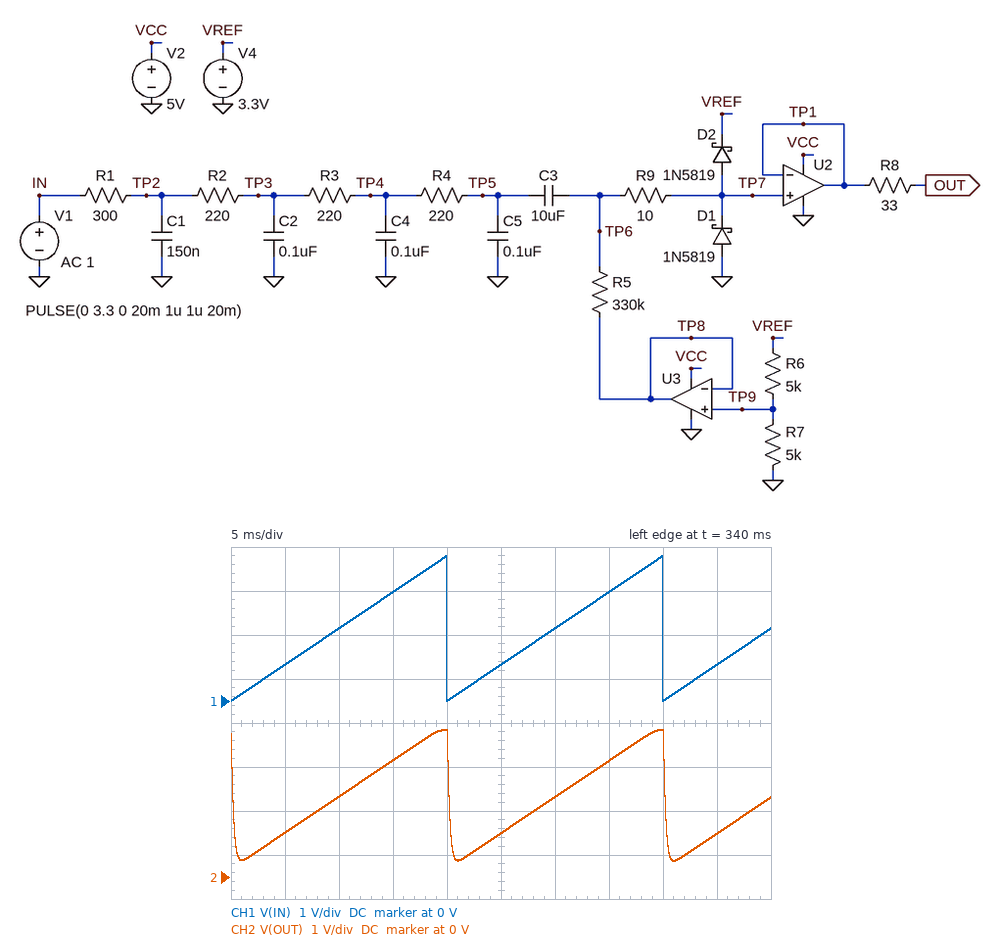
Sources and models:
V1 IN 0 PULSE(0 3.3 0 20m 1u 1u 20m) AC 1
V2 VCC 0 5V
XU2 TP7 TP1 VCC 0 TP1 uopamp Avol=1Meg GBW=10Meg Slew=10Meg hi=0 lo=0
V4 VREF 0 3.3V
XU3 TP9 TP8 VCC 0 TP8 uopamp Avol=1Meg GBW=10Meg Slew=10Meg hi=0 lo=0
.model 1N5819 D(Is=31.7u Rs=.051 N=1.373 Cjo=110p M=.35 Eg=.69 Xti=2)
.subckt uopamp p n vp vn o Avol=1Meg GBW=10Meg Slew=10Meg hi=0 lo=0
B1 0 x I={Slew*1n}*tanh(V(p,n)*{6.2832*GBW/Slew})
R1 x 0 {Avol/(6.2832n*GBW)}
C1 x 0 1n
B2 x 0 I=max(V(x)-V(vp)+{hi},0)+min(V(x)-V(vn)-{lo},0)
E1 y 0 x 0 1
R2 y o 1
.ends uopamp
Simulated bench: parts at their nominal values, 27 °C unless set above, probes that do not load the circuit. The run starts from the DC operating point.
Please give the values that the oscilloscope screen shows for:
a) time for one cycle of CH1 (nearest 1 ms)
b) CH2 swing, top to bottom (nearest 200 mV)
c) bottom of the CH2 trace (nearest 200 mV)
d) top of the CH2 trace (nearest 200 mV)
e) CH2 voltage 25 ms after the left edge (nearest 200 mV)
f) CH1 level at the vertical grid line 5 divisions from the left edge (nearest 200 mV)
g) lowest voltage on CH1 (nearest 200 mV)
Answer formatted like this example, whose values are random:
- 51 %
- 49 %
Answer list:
- 20 ms
- 3.0 V
- 400 mV
- 3.4 V
- 1.0 V
- 800 mV
- 0 V
